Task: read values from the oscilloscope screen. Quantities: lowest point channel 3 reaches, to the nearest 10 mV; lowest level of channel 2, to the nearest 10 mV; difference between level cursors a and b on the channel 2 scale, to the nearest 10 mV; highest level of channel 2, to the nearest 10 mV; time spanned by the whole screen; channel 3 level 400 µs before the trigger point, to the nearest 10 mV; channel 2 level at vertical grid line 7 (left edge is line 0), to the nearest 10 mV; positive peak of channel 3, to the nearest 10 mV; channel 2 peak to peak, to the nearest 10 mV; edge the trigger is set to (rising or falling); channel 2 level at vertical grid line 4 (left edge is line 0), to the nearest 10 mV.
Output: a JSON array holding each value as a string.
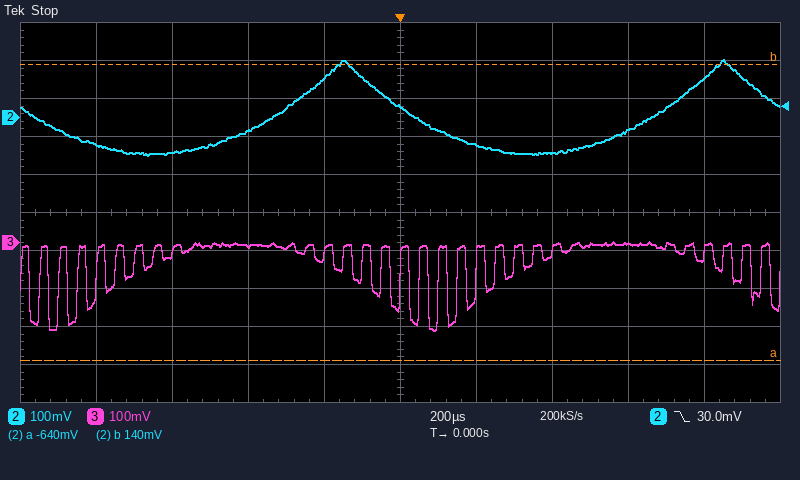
["-230 mV", "-100 mV", "780 mV", "150 mV", "2 ms", "-10 mV", "-90 mV", "0 mV", "250 mV", "falling", "100 mV"]
